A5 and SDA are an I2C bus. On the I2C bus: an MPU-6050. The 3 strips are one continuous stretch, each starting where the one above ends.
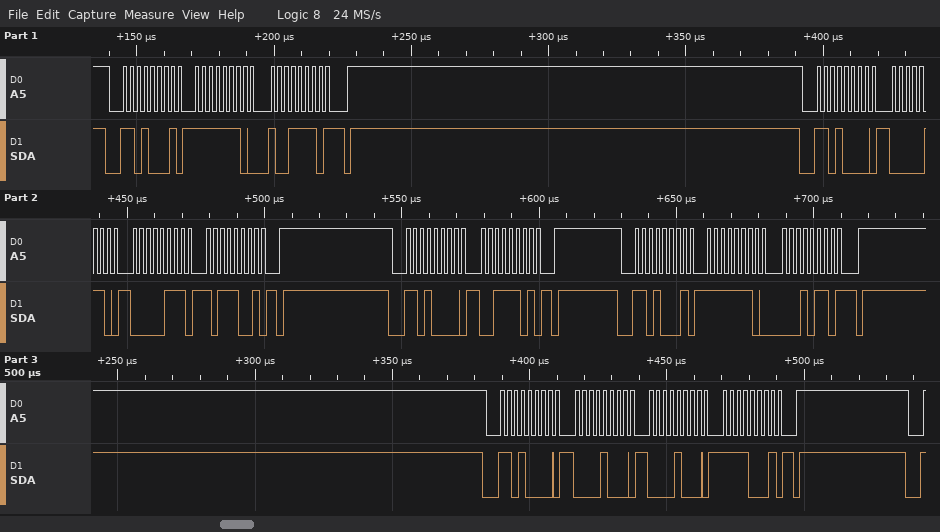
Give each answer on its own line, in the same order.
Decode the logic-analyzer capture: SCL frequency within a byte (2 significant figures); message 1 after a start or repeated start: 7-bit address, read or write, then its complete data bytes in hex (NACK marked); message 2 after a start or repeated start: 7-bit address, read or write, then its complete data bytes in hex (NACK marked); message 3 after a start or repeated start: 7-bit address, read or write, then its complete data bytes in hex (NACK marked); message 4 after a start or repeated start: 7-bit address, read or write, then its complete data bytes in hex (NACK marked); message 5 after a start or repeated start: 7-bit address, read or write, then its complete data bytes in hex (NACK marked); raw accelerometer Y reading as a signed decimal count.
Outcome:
400 kHz
0x68 read: FE 9E NACK
0x68 write: 06 07 B9
0x68 write: 3D
0x68 read: FE 16 NACK
0x68 write: 08 08 F1
-490
